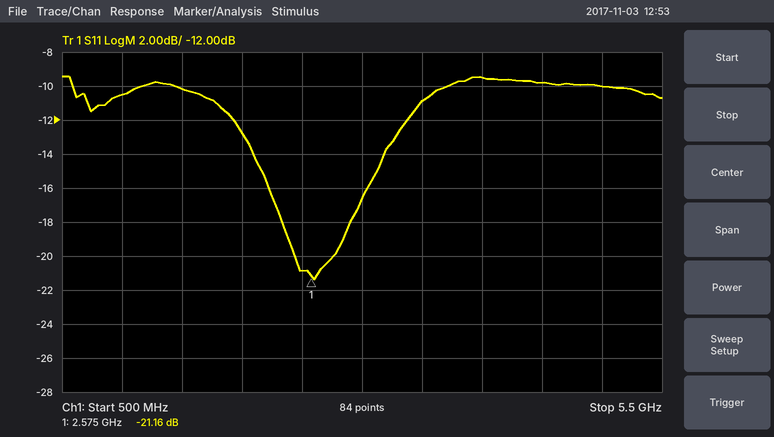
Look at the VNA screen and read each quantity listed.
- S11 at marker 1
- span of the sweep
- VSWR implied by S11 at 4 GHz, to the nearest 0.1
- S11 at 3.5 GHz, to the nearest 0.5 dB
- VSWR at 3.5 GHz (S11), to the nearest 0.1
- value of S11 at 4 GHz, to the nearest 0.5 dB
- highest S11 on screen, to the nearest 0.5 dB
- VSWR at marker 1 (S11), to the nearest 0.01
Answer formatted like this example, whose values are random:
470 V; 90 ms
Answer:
-21.16 dB; 5 GHz; 2.0; -11.0 dB; 1.8; -9.5 dB; -9.5 dB; 1.19
